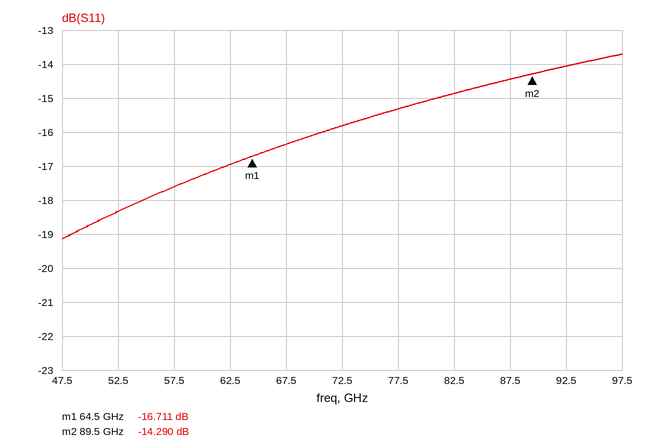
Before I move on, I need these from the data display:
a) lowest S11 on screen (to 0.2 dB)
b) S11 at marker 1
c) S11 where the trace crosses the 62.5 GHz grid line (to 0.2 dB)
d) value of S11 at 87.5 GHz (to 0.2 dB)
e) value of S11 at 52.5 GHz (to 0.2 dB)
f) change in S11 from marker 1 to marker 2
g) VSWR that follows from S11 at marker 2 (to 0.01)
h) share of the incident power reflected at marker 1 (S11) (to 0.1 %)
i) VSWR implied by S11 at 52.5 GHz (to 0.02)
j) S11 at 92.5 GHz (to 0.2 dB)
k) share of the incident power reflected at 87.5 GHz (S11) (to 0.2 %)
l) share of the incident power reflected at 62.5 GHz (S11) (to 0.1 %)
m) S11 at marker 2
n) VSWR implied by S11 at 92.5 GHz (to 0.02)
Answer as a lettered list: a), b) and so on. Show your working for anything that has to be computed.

a) -19.2 dB
b) -16.711 dB
c) -17.0 dB
d) -14.4 dB
e) -18.4 dB
f) -14.29 − (-16.711) = 2.421 dB
g) (1 + 0.1930)/(1 − 0.1930) ≈ 1.48
h) 10^(-16.711/10) ≈ 2.1 %
i) |Γ| = 10^(-18.4/20) = 0.1202; VSWR = (1 + 0.1202)/(1 − 0.1202) ≈ 1.27, so 1.28 to the nearest 0.02
j) -14.0 dB
k) 10^(-14.4/10) ≈ 3.6 %
l) 10^(-17/10) ≈ 2.0 %
m) -14.290 dB
n) |Γ| = 10^(-14/20) = 0.1995; VSWR = (1 + 0.1995)/(1 − 0.1995) ≈ 1.50
